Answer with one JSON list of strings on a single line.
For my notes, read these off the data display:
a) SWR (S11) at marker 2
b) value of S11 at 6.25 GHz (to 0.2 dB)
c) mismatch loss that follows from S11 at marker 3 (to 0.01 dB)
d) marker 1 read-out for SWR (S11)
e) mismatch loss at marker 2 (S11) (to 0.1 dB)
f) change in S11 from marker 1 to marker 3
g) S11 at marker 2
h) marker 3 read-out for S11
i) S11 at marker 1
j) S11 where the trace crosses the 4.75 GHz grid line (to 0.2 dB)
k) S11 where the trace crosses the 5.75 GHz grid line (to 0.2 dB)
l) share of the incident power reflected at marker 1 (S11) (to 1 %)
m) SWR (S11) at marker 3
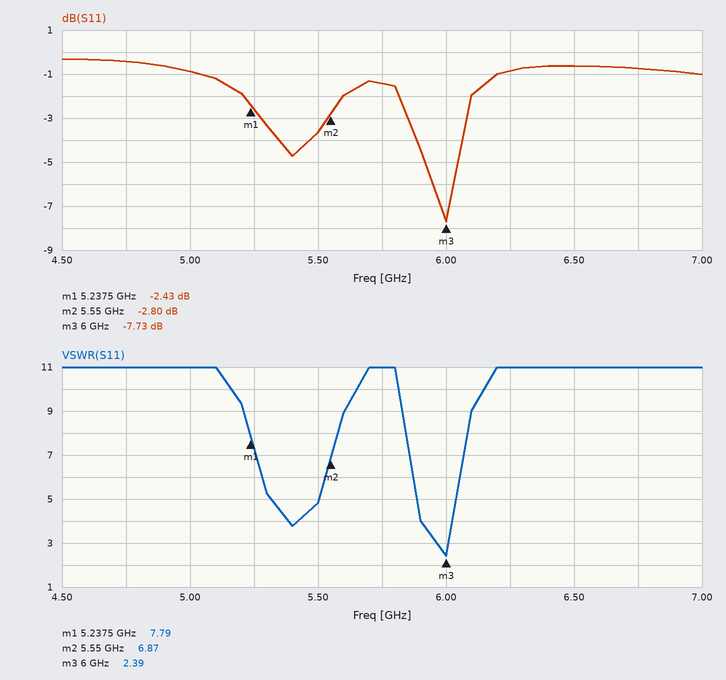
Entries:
["6.87", "-0.8 dB", "0.80 dB", "7.79", "3.2 dB", "-5.30 dB", "-2.80 dB", "-7.73 dB", "-2.43 dB", "-0.4 dB", "-1.4 dB", "57 %", "2.39"]
